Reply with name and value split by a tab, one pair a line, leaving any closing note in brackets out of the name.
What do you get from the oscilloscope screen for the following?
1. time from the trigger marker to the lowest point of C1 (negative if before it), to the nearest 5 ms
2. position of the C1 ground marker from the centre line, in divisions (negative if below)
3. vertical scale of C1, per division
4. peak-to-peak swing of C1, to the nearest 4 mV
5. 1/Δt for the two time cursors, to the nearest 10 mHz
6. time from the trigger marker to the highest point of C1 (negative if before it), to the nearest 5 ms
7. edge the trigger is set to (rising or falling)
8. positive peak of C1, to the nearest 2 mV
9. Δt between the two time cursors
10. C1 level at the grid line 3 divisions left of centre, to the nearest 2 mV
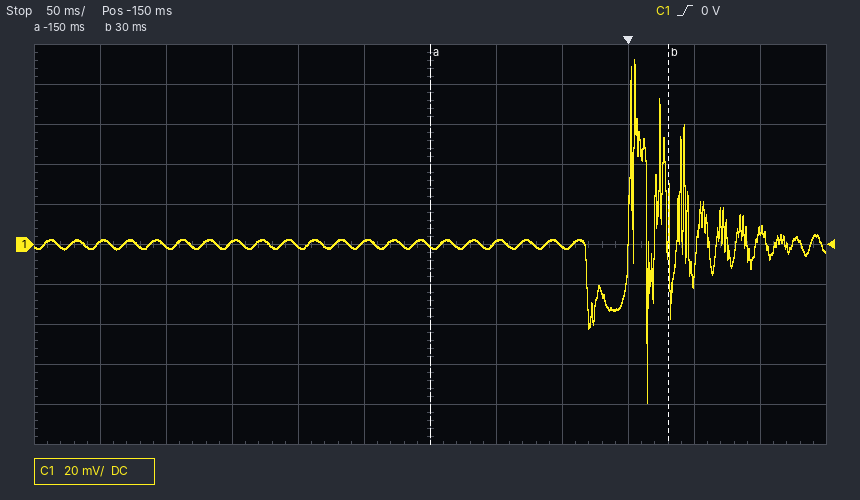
time from the trigger marker to the lowest point of C1 (negative if before it), to the nearest 5 ms	+15 ms
position of the C1 ground marker from the centre line, in divisions	0.0 div
vertical scale of C1, per division	20 mV
peak-to-peak swing of C1, to the nearest 4 mV	172 mV
1/Δt for the two time cursors, to the nearest 10 mHz	5.56 Hz
time from the trigger marker to the highest point of C1 (negative if before it), to the nearest 5 ms	+5 ms
edge the trigger is set to	rising
positive peak of C1, to the nearest 2 mV	92 mV
Δt between the two time cursors	180 ms
C1 level at the grid line 3 divisions left of centre, to the nearest 2 mV	2 mV
